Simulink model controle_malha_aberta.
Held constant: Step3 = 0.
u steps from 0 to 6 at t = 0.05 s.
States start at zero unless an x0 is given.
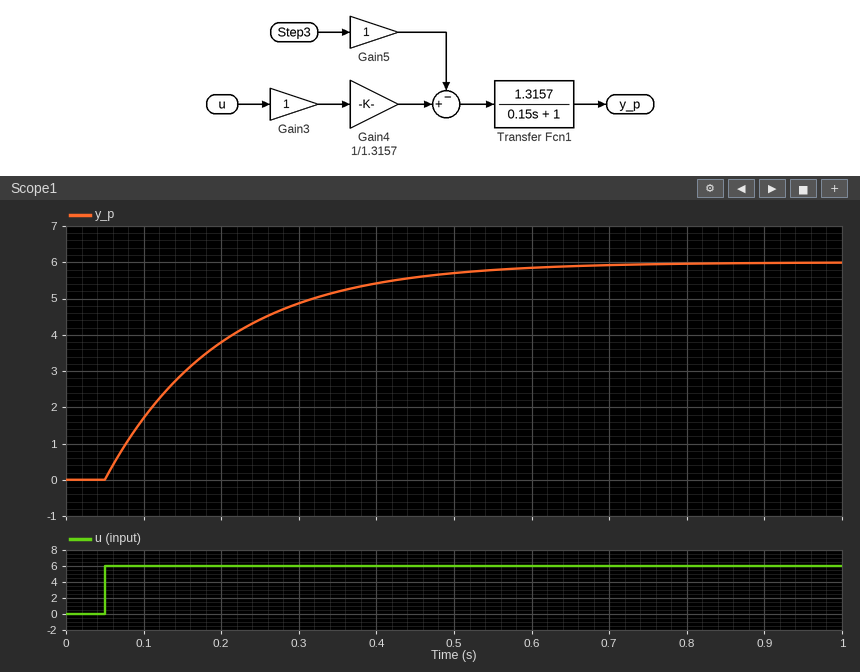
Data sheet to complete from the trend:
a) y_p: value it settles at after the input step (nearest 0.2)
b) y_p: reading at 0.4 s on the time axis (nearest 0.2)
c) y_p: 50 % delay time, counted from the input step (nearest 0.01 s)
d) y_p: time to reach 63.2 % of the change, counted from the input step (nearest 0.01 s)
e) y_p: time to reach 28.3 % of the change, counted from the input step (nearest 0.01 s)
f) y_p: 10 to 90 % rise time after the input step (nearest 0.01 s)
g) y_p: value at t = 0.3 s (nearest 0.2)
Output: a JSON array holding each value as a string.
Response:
["6.0", "5.4", "0.10 s", "0.15 s", "0.05 s", "0.33 s", "4.8"]
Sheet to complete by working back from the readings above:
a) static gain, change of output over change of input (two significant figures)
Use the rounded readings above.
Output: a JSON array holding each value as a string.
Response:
["1.0"]
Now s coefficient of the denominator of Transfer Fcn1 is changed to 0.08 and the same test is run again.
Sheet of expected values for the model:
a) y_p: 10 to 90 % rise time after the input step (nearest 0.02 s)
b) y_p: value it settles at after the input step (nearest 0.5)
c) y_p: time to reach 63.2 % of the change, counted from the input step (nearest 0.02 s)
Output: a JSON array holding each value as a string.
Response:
["0.18 s", "6.0", "0.08 s"]
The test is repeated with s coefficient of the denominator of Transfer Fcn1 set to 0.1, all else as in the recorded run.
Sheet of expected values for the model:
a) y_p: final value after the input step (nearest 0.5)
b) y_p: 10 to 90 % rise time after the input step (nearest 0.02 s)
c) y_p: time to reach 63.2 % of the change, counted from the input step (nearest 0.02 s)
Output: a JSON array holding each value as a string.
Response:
["6.0", "0.22 s", "0.10 s"]
